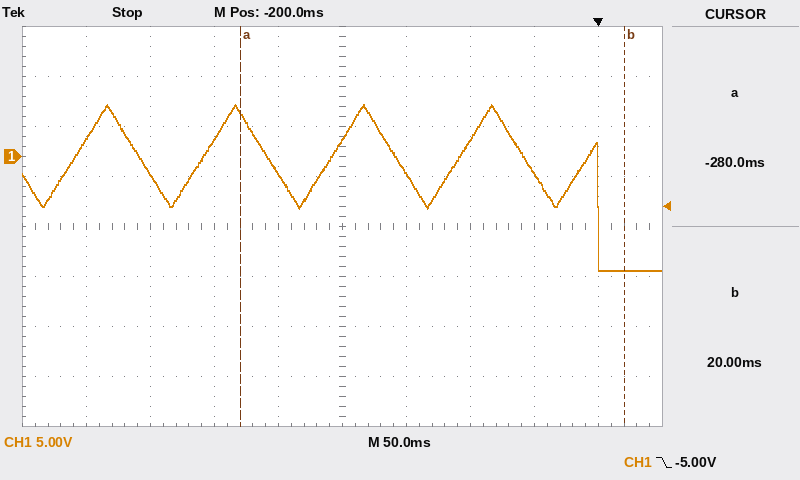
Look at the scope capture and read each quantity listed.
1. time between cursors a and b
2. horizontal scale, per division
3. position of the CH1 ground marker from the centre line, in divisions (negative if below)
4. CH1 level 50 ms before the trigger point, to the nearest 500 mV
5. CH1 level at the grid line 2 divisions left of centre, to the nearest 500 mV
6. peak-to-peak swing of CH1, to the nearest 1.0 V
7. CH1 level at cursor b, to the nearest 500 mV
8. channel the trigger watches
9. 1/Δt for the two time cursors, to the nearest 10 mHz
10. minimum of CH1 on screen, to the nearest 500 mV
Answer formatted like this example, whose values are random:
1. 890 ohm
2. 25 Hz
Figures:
1. 300 ms
2. 50 ms
3. +1.4 div
4. -1.5 V
5. 1.5 V
6. 17.0 V
7. -11.5 V
8. CH1
9. 3.33 Hz
10. -11.5 V
